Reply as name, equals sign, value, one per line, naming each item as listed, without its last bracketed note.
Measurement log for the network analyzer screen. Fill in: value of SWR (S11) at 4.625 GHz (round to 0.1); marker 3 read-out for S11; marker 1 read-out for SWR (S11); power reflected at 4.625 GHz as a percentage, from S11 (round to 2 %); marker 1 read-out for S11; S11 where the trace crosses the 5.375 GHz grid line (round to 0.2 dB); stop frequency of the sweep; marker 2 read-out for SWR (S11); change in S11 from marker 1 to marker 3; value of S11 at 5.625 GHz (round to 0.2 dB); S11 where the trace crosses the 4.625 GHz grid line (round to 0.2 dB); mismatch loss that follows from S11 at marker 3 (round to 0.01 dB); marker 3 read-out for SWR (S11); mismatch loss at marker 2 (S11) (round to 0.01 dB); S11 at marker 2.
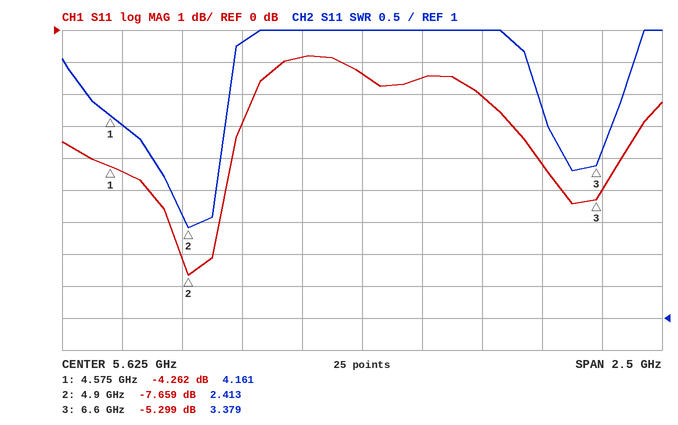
value of SWR (S11) at 4.625 GHz = 4.0
marker 3 read-out for S11 = -5.299 dB
marker 1 read-out for SWR = 4.161
power reflected at 4.625 GHz as a percentage, from S11 = 36 %
marker 1 read-out for S11 = -4.262 dB
S11 where the trace crosses the 5.375 GHz grid line = -0.8 dB
stop frequency of the sweep = 6.875 GHz
marker 2 read-out for SWR = 2.413
change in S11 from marker 1 to marker 3 = -1.037 dB
value of S11 at 5.625 GHz = -1.4 dB
S11 where the trace crosses the 4.625 GHz grid line = -4.4 dB
mismatch loss that follows from S11 at marker 3 = 1.52 dB
marker 3 read-out for SWR = 3.379
mismatch loss at marker 2 (S11) = 0.82 dB
S11 at marker 2 = -7.659 dB
